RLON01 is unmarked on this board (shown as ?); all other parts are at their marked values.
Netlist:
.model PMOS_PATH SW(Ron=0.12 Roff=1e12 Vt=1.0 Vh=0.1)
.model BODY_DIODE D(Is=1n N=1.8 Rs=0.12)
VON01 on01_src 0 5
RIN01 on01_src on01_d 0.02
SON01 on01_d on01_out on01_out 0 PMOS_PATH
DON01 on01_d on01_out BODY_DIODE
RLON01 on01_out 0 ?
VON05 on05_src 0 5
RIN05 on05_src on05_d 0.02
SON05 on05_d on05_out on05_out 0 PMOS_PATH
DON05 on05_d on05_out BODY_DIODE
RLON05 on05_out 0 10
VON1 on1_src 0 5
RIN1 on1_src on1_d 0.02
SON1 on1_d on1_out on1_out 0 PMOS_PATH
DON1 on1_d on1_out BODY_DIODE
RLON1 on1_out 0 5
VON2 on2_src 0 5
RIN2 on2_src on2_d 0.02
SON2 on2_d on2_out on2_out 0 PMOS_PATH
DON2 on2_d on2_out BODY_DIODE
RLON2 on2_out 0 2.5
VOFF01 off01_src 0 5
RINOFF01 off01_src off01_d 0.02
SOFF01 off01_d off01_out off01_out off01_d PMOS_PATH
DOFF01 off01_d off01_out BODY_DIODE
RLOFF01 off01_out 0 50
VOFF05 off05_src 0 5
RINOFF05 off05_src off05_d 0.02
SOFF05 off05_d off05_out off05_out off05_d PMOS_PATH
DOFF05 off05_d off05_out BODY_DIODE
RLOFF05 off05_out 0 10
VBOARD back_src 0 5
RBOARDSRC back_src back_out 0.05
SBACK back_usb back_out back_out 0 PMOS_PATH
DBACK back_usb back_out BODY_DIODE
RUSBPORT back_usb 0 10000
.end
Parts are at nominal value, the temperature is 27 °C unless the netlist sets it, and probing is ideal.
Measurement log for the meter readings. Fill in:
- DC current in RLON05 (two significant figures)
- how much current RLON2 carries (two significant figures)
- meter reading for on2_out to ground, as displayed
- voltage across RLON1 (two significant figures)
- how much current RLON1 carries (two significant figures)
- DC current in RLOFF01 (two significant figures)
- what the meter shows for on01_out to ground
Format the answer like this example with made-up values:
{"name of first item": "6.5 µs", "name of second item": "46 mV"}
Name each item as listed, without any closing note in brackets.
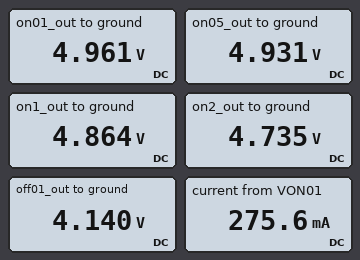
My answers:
{"DC current in RLON05": "490 mA", "how much current RLON2 carries": "1.9 A", "meter reading for on2_out to ground, as displayed": "4.735 V", "voltage across RLON1": "4.9 V", "how much current RLON1 carries": "970 mA", "DC current in RLOFF01": "83 mA", "what the meter shows for on01_out to ground": "4.961 V"}
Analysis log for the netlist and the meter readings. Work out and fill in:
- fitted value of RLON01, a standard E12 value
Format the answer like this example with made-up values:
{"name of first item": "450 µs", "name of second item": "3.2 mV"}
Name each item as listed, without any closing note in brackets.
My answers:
{"fitted value of RLON01, a standard E12 value": "18 Ω"}
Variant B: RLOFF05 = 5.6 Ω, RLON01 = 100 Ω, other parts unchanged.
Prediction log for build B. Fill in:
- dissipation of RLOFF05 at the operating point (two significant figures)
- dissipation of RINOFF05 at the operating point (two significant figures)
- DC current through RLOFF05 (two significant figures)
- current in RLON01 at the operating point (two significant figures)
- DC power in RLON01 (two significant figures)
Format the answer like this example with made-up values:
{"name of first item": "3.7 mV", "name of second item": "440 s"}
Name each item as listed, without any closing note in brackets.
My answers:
{"dissipation of RLOFF05 at the operating point": "2.8 W", "dissipation of RINOFF05 at the operating point": "10 mW", "DC current through RLOFF05": "710 mA", "current in RLON01 at the operating point": "50 mA", "DC power in RLON01": "250 mW"}
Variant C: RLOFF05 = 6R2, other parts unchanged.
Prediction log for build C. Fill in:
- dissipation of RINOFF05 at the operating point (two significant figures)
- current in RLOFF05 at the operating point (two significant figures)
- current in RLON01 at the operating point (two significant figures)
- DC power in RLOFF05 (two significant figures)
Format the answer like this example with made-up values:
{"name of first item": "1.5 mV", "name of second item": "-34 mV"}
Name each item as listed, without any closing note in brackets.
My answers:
{"dissipation of RINOFF05 at the operating point": "8.2 mW", "current in RLOFF05 at the operating point": "640 mA", "current in RLON01 at the operating point": "280 mA", "DC power in RLOFF05": "2.5 W"}
